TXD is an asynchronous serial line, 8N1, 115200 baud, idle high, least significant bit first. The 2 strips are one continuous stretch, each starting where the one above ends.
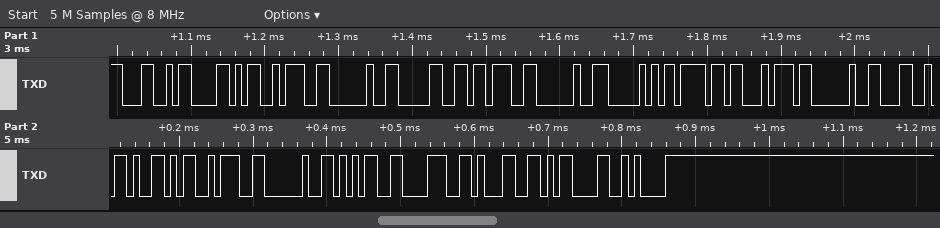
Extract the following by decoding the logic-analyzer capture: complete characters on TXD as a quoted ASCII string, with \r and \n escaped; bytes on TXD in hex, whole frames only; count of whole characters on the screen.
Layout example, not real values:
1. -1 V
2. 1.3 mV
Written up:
1. "LX: 0; Pot LY: 581\r\n"
2. 4C 58 3A 20 30 3B 20 50 6F 74 20 4C 59 3A 20 35 38 31 0D 0A
3. 20
